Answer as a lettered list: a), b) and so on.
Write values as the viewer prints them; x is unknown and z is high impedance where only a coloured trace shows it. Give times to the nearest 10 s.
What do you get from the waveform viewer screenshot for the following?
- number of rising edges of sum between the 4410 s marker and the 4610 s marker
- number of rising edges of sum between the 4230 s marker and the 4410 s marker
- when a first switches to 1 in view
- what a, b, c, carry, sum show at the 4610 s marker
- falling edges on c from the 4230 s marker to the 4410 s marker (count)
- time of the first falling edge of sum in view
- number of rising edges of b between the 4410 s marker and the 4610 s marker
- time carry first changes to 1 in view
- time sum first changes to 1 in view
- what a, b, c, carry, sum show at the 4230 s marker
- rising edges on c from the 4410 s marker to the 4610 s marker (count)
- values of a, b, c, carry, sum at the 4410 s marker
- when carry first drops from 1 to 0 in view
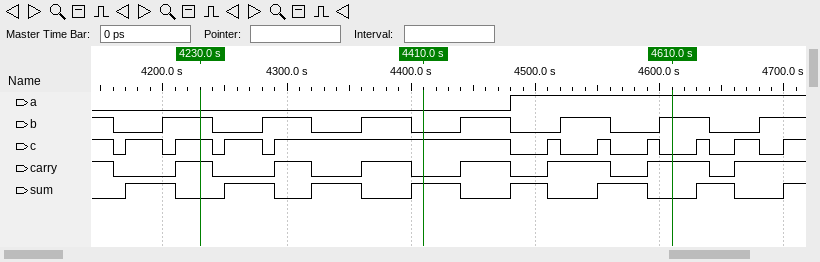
a) 2
b) 3
c) 4480 s
d) a=1, b=1, c=0, carry=1, sum=0
e) 2
f) 4210 s
g) 3
h) 4210 s
i) 4170 s
j) a=0, b=1, c=1, carry=1, sum=0
k) 3
l) a=0, b=0, c=1, carry=0, sum=1
m) 4160 s
